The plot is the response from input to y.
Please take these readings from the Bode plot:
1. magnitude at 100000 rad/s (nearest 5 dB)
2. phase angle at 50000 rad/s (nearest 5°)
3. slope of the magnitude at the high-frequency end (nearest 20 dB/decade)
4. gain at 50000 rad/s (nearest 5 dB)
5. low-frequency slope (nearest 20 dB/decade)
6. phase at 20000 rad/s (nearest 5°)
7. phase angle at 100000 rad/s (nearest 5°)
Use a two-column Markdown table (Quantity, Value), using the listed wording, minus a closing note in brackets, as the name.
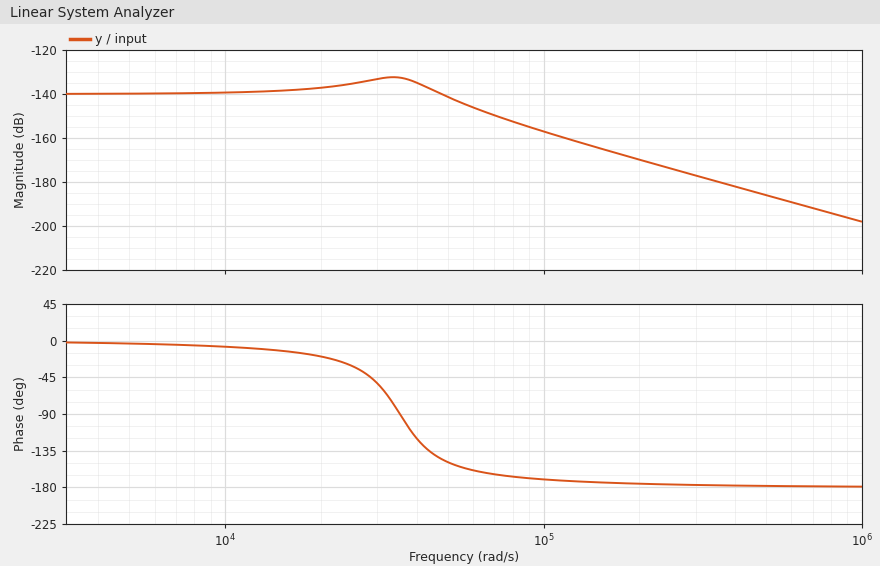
| Quantity | Value |
|---|---|
| magnitude at 100000 rad/s | -155 dB |
| phase angle at 50000 rad/s | -150° |
| slope of the magnitude at the high-frequency end | -40 dB/decade |
| gain at 50000 rad/s | -140 dB |
| low-frequency slope | 0 dB/decade |
| phase at 20000 rad/s | -20° |
| phase angle at 100000 rad/s | -170° |
